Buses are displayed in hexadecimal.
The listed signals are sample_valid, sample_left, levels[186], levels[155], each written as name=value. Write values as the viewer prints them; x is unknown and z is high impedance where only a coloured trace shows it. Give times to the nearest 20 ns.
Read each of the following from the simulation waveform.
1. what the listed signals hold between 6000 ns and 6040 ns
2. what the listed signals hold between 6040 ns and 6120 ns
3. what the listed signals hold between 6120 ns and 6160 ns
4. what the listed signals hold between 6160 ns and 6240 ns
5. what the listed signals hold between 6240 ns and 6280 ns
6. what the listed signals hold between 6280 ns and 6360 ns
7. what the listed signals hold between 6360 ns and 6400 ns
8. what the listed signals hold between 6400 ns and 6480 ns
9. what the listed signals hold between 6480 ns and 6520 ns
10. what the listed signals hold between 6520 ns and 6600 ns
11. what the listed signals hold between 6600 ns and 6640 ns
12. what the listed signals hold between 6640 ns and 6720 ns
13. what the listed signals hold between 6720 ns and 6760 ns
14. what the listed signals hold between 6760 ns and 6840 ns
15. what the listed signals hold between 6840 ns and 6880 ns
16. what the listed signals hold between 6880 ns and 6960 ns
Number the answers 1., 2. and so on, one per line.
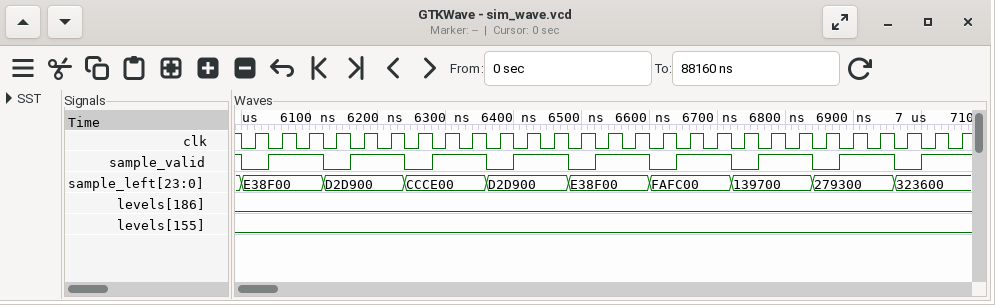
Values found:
1. sample_valid=0, sample_left=E38F00, levels[186]=0, levels[155]=0
2. sample_valid=1, sample_left=E38F00, levels[186]=0, levels[155]=0
3. sample_valid=0, sample_left=D2D900, levels[186]=0, levels[155]=0
4. sample_valid=1, sample_left=D2D900, levels[186]=0, levels[155]=0
5. sample_valid=0, sample_left=CCCE00, levels[186]=0, levels[155]=0
6. sample_valid=1, sample_left=CCCE00, levels[186]=0, levels[155]=0
7. sample_valid=0, sample_left=D2D900, levels[186]=0, levels[155]=0
8. sample_valid=1, sample_left=D2D900, levels[186]=0, levels[155]=0
9. sample_valid=0, sample_left=E38F00, levels[186]=0, levels[155]=0
10. sample_valid=1, sample_left=E38F00, levels[186]=0, levels[155]=0
11. sample_valid=0, sample_left=FAFC00, levels[186]=0, levels[155]=0
12. sample_valid=1, sample_left=FAFC00, levels[186]=0, levels[155]=0
13. sample_valid=0, sample_left=139700, levels[186]=0, levels[155]=0
14. sample_valid=1, sample_left=139700, levels[186]=0, levels[155]=0
15. sample_valid=0, sample_left=279300, levels[186]=0, levels[155]=0
16. sample_valid=1, sample_left=279300, levels[186]=0, levels[155]=0
